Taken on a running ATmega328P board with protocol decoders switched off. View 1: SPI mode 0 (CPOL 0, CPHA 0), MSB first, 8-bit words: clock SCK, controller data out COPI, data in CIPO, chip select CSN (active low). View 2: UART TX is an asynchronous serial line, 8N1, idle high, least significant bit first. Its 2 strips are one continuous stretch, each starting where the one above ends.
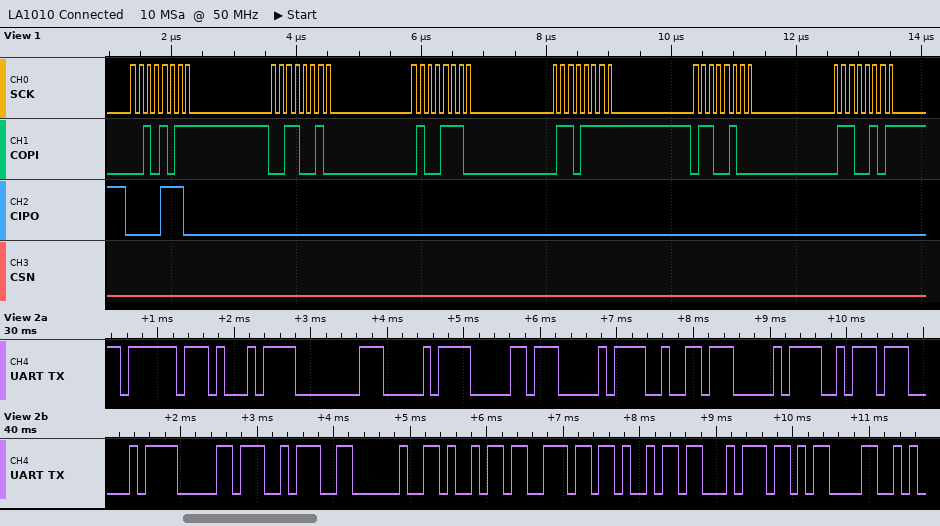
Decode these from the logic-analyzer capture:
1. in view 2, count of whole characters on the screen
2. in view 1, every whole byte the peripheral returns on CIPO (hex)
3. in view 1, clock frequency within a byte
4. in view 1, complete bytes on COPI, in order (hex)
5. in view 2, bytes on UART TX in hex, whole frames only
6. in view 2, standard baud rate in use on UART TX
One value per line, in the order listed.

18
0E 00 00 00 00 00
8 MHz
2B 32 4E 6F 64 65
BF D1 80 D0 B0 D0 B2 D0 BA D0 B0 3A 20 69 6E 69 74 0D
9600 baud
